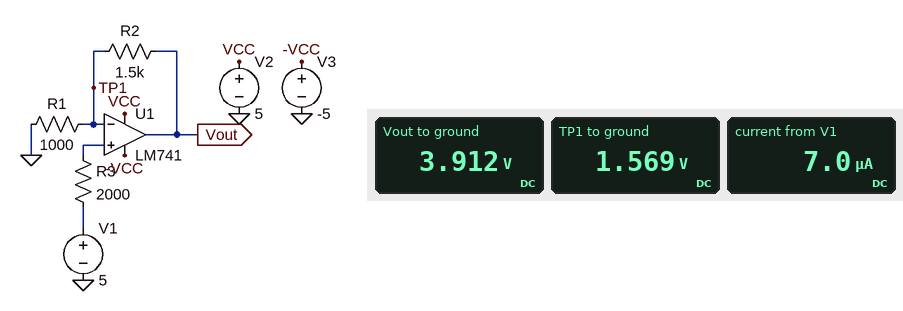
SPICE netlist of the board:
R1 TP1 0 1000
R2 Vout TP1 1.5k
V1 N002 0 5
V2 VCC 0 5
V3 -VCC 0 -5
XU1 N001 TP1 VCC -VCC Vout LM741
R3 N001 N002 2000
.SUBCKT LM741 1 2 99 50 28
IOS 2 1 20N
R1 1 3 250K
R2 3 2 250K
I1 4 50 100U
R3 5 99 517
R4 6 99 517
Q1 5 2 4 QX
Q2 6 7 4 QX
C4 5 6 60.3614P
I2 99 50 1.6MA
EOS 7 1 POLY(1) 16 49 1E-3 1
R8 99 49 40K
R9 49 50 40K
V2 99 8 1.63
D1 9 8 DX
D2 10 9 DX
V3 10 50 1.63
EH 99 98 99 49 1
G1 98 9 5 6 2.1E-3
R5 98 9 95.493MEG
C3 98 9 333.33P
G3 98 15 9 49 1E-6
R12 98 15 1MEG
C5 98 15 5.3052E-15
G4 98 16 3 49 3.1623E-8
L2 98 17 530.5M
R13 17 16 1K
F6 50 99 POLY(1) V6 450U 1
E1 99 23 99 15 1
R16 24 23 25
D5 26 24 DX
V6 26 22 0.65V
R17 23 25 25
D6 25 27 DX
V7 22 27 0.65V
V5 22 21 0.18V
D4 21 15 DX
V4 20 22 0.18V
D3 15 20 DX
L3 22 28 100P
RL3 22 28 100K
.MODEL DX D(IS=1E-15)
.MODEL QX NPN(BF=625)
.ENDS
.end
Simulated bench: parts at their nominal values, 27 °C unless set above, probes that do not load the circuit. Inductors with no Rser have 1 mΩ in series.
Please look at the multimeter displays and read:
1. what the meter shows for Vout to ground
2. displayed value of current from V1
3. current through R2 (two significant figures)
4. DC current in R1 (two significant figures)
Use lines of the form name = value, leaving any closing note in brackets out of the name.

what the meter shows for Vout to ground = 3.912 V
displayed value of current from V1 = 7.0 µA
current through R2 = 1.6 mA
DC current in R1 = 1.6 mA
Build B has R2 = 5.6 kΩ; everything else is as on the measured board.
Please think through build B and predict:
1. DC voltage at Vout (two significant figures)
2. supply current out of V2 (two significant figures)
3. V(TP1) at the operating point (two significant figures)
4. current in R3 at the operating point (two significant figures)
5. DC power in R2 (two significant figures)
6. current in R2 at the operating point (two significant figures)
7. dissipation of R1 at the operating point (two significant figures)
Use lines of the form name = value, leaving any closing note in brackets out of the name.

DC voltage at Vout = 4.0 V
supply current out of V2 = 2.0 mA
V(TP1) at the operating point = 610 mV
current in R3 at the operating point = 8.9 µA
DC power in R2 = 2.0 mW
current in R2 at the operating point = 600 µA
dissipation of R1 at the operating point = 370 µW
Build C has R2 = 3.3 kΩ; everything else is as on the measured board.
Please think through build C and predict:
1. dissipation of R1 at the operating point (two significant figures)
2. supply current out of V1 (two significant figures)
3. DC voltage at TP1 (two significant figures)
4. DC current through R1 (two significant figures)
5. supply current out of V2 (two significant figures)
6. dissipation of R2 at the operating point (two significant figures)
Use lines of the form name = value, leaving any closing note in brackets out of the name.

dissipation of R1 at the operating point = 850 µW
supply current out of V1 = 8.3 µA
DC voltage at TP1 = 920 mV
DC current through R1 = 920 µA
supply current out of V2 = 2.3 mA
dissipation of R2 at the operating point = 2.8 mW
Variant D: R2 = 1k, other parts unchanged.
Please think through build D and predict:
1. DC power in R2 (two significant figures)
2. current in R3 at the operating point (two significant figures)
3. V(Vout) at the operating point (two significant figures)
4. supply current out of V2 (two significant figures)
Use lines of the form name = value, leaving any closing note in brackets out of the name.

DC power in R2 = 3.8 mW
current in R3 at the operating point = 6.2 µA
V(Vout) at the operating point = 3.9 V
supply current out of V2 = 3.3 mA
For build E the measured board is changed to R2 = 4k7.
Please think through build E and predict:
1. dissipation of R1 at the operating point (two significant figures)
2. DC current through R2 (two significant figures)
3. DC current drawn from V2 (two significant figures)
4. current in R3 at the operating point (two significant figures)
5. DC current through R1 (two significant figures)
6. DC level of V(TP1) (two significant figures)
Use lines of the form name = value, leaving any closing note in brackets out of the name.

dissipation of R1 at the operating point = 490 µW
DC current through R2 = 690 µA
DC current drawn from V2 = 2.1 mA
current in R3 at the operating point = 8.7 µA
DC current through R1 = 700 µA
DC level of V(TP1) = 700 mV
